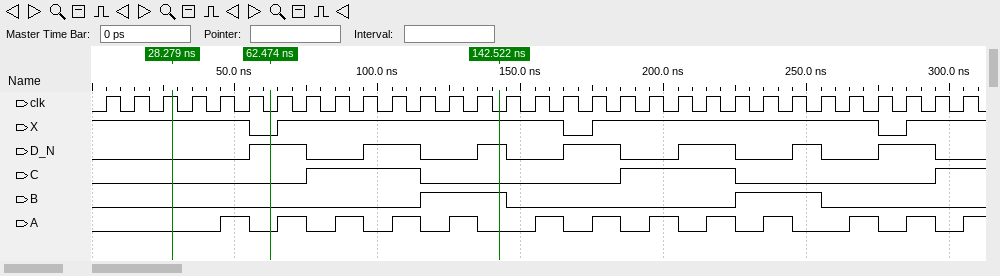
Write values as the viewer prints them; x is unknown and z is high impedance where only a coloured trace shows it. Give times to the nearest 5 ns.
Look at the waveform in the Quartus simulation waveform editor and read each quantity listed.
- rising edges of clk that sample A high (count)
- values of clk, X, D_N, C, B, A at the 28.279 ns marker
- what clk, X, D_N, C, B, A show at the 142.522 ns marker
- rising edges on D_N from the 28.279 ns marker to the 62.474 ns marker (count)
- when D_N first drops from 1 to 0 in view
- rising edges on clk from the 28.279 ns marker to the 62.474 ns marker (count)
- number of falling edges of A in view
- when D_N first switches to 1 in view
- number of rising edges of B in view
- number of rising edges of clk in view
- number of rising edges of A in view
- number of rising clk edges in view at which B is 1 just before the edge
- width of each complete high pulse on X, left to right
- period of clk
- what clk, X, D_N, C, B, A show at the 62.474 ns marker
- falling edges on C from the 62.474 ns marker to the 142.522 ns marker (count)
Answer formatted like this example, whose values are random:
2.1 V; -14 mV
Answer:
12; clk=1, X=1, D_N=0, C=0, B=0, A=0; clk=0, X=1, D_N=1, C=0, B=1, A=0; 1; 75 ns; 3; 12; 55 ns; 2; 31; 13; 6; 100 ns, 100 ns; 10 ns; clk=0, X=0, D_N=1, C=0, B=0, A=0; 1
